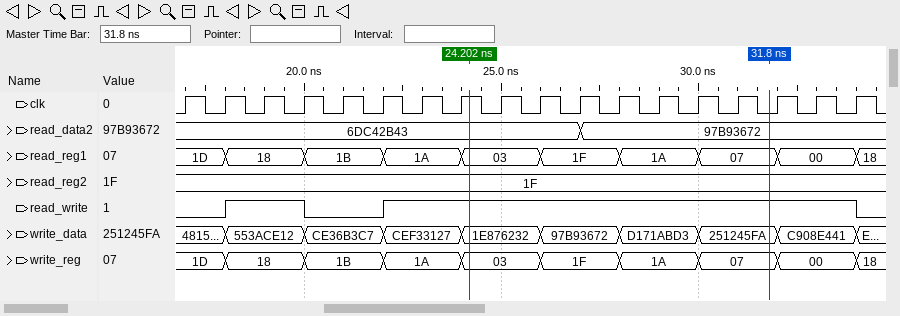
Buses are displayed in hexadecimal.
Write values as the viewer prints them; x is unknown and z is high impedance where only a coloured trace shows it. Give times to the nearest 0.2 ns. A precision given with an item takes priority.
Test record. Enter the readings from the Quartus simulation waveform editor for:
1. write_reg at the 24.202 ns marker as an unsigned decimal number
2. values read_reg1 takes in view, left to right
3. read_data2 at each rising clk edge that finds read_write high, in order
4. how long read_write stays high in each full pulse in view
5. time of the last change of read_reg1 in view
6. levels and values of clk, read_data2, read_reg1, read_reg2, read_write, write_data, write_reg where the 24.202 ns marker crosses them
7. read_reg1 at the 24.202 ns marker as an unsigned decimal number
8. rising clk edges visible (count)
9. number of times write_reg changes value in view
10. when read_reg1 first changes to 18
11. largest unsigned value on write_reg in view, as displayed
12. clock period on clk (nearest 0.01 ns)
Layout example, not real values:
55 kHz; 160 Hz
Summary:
3; 1D, 18, 1B, 1A, 03, 1F, 1A, 07, 00, 18; 6DC42B43, 6DC42B43, 6DC42B43, 6DC42B43, 6DC42B43, 6DC42B43, 6DC42B43, 97B93672, 97B93672, 97B93672, 97B93672, 97B93672, 97B93672, 97B93672; 2 ns, 12 ns; 34 ns; clk=1, read_data2=6DC42B43, read_reg1=03, read_reg2=1F, read_write=1, write_data=1E876232, write_reg=03; 3; 18; 9; 18 ns; 1F; 1 ns
